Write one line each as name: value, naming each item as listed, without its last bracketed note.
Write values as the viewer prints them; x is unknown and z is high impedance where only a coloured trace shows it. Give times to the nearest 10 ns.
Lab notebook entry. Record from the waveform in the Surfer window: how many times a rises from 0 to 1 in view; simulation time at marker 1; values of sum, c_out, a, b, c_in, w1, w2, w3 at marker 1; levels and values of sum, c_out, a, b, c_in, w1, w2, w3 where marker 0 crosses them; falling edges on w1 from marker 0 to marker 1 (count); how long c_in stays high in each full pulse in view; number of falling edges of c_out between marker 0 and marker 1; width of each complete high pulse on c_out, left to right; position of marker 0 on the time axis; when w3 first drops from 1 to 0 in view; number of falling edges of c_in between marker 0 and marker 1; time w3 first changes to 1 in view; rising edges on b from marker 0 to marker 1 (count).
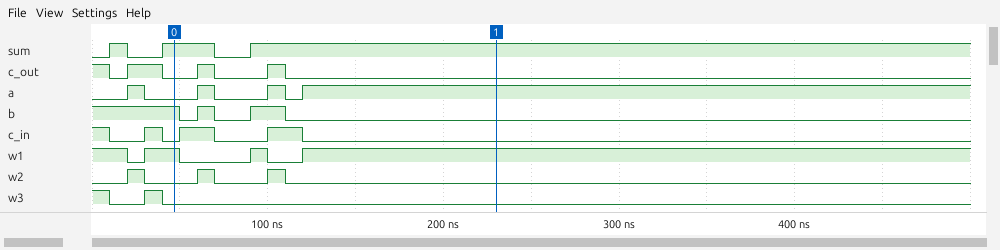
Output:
how many times a rises from 0 to 1 in view: 4
simulation time at marker 1: 230 ns
values of sum, c_out, a, b, c_in, w1, w2, w3 at marker 1: sum=1, c_out=0, a=1, b=0, c_in=0, w1=1, w2=0, w3=0
levels and values of sum, c_out, a, b, c_in, w1, w2, w3 where marker 0 crosses them: sum=1, c_out=0, a=0, b=1, c_in=0, w1=1, w2=0, w3=0
falling edges on w1 from marker 0 to marker 1: 2
how long c_in stays high in each full pulse in view: 10 ns, 20 ns, 20 ns
number of falling edges of c_out between marker 0 and marker 1: 2
width of each complete high pulse on c_out, left to right: 20 ns, 10 ns, 10 ns
position of marker 0 on the time axis: 50 ns
when w3 first drops from 1 to 0 in view: 10 ns
number of falling edges of c_in between marker 0 and marker 1: 2
time w3 first changes to 1 in view: 30 ns
rising edges on b from marker 0 to marker 1: 2
